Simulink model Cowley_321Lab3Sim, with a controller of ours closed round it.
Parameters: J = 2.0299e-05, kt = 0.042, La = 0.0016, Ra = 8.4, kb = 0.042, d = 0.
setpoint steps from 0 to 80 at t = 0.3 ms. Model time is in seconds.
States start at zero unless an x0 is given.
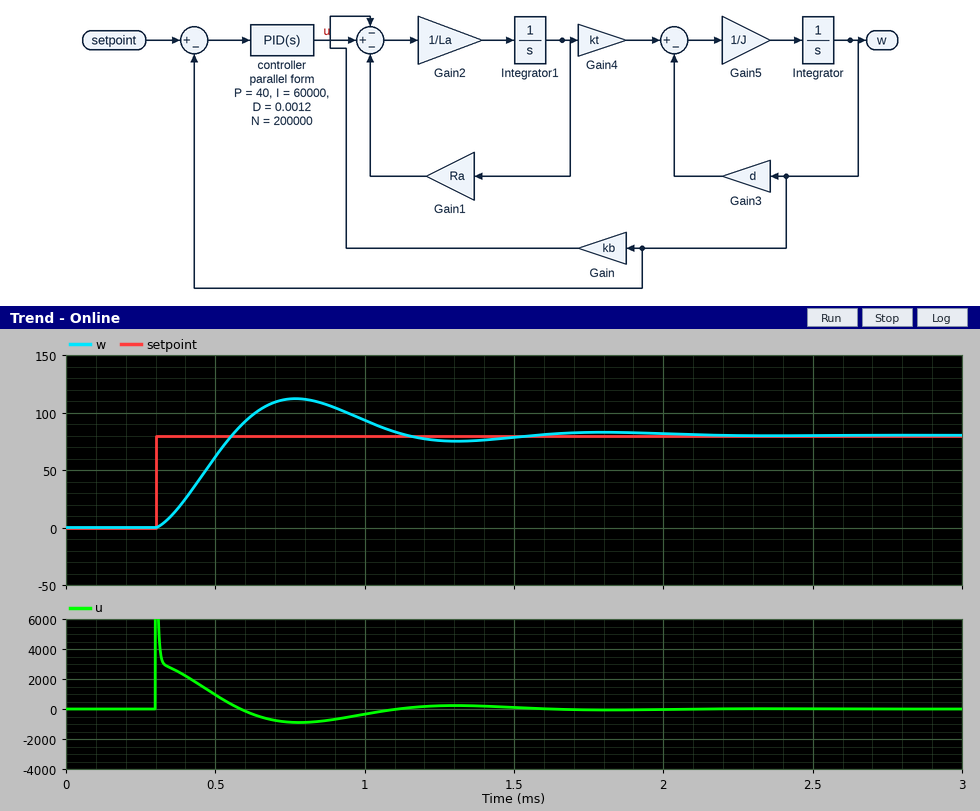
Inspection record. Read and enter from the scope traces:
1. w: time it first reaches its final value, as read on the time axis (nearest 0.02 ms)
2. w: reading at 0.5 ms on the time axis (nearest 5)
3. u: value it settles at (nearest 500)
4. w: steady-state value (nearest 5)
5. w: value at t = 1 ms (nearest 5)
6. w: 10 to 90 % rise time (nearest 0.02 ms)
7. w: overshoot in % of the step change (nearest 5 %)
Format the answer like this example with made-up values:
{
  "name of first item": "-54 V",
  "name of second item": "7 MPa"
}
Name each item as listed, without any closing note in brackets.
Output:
{
  "w: time it first reaches its final value, as read on the time axis": "0.56 ms",
  "w: reading at 0.5 ms on the time axis": "60",
  "u: value it settles at": "0",
  "w: steady-state value": "80",
  "w: value at t = 1 ms": "95",
  "w: 10 to 90 % rise time": "0.18 ms",
  "w: overshoot in % of the step change": "40 %"
}
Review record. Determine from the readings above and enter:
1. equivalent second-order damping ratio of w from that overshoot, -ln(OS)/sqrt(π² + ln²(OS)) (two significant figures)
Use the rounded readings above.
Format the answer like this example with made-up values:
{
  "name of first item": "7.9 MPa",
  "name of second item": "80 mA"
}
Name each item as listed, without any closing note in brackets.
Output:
{
  "equivalent second-order damping ratio of w from that overshoot, -ln(OS)/sqrt(π² + ln²(OS))": "0.28"
}
